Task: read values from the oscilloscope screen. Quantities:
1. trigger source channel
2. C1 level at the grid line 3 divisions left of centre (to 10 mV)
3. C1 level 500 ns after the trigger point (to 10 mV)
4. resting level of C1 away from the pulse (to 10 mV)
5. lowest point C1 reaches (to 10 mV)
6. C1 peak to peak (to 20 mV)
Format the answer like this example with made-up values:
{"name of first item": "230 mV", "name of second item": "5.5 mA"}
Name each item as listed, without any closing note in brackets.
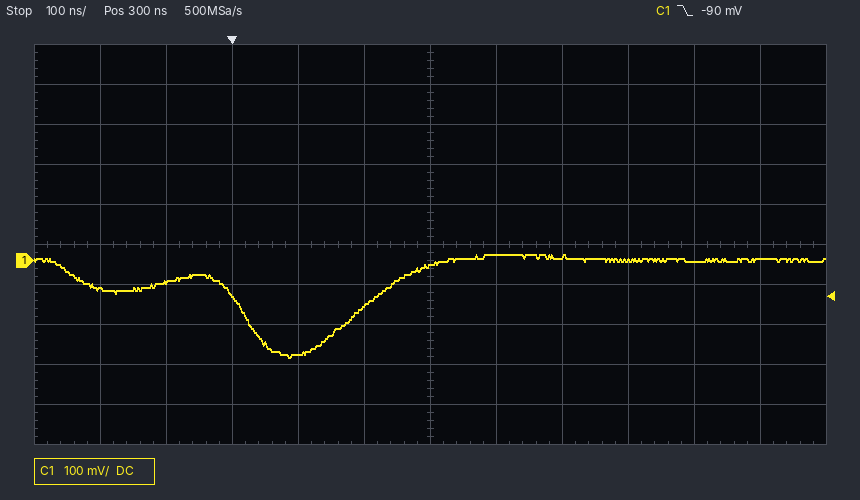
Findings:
{"trigger source channel": "C1", "C1 level at the grid line 3 divisions left of centre": "-90 mV", "C1 level 500 ns after the trigger point": "10 mV", "resting level of C1 away from the pulse": "0 mV", "lowest point C1 reaches": "-240 mV", "C1 peak to peak": "260 mV"}
